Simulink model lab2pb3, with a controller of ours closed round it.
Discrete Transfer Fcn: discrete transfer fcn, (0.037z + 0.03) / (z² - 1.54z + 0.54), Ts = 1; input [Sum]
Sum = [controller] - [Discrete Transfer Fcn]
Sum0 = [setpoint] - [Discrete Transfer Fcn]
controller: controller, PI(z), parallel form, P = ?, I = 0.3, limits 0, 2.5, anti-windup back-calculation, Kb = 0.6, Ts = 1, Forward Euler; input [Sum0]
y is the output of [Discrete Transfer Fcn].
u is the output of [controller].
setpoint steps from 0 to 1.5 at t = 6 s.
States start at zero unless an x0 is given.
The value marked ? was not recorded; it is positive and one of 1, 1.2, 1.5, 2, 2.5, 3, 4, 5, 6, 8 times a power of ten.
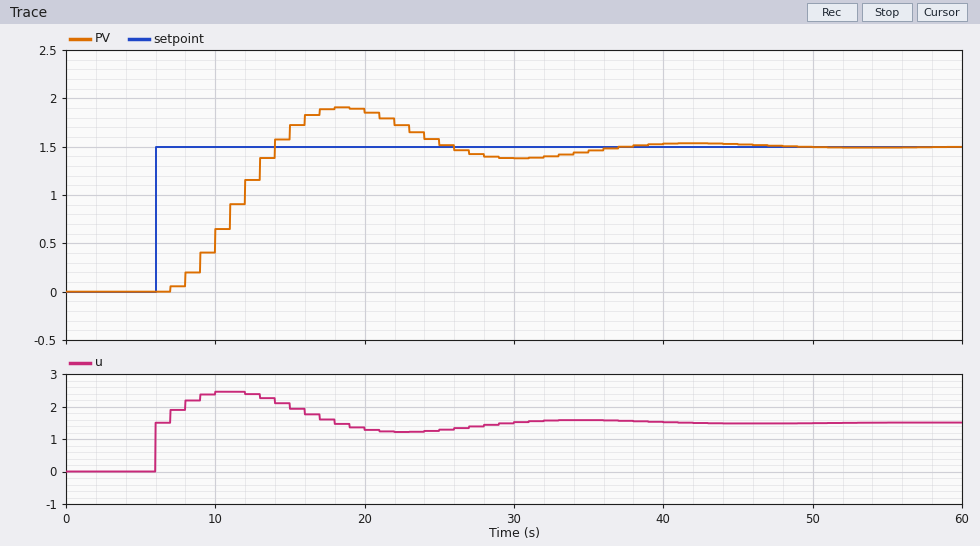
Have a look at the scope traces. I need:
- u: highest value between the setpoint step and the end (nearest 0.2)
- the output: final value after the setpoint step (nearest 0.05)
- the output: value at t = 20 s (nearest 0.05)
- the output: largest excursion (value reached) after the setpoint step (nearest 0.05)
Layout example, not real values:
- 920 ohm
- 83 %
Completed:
- 2.4
- 1.50
- 1.85
- 1.90
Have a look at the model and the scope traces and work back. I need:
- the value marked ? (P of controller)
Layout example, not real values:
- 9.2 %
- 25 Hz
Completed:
- 1
